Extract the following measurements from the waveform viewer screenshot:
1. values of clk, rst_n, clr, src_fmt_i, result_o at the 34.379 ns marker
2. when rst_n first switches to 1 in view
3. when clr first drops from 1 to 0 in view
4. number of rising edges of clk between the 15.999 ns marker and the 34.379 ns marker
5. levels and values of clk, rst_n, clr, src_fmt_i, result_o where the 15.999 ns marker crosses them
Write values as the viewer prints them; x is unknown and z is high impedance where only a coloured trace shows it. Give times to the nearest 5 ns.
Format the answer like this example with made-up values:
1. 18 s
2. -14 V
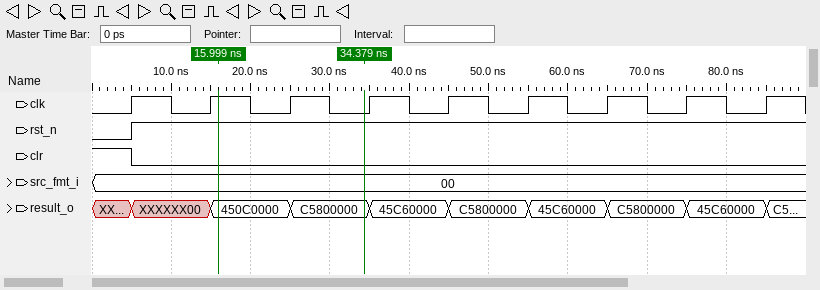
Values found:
1. clk=0, rst_n=1, clr=0, src_fmt_i=00, result_o=C5800000
2. 5 ns
3. 5 ns
4. 1
5. clk=1, rst_n=1, clr=0, src_fmt_i=00, result_o=450C0000
